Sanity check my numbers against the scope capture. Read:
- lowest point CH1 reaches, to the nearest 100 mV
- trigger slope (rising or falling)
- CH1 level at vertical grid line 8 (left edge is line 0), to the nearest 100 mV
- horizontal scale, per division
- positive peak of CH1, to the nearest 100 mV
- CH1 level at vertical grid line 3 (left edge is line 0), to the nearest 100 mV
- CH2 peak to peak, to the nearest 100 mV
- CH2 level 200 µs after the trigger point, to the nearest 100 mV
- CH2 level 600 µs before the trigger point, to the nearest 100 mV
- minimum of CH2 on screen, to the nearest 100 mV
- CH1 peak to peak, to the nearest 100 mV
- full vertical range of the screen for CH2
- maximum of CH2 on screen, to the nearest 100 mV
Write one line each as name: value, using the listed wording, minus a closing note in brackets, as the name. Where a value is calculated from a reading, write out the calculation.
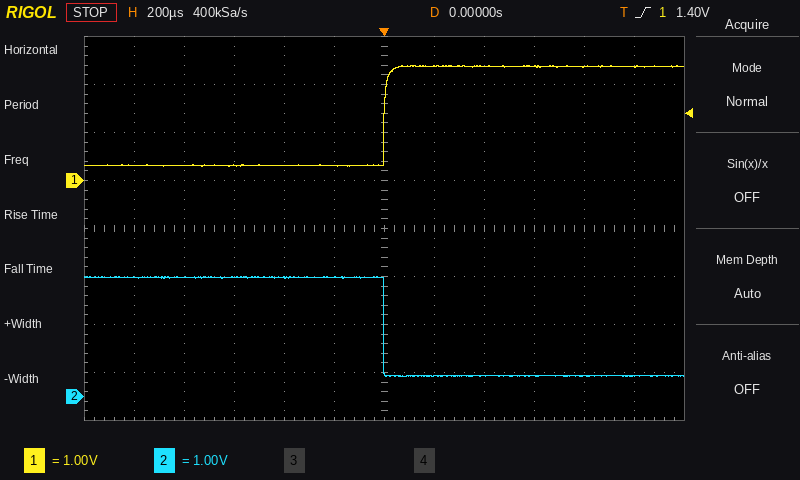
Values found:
lowest point CH1 reaches, to the nearest 100 mV: 300 mV
trigger slope: rising
CH1 level at vertical grid line 8 (left edge is line 0), to the nearest 100 mV: 2.4 V
horizontal scale, per division: 200 µs
positive peak of CH1, to the nearest 100 mV: 2.4 V
CH1 level at vertical grid line 3 (left edge is line 0), to the nearest 100 mV: 300 mV
CH2 peak to peak, to the nearest 100 mV: 2.5 V − (400 mV) = 2.1 V
CH2 level 200 µs after the trigger point, to the nearest 100 mV: 400 mV
CH2 level 600 µs before the trigger point, to the nearest 100 mV: 2.5 V
minimum of CH2 on screen, to the nearest 100 mV: 400 mV
CH1 peak to peak, to the nearest 100 mV: 2.4 V − (300 mV) = 2.1 V
full vertical range of the screen for CH2: 8 V
maximum of CH2 on screen, to the nearest 100 mV: 2.5 V
